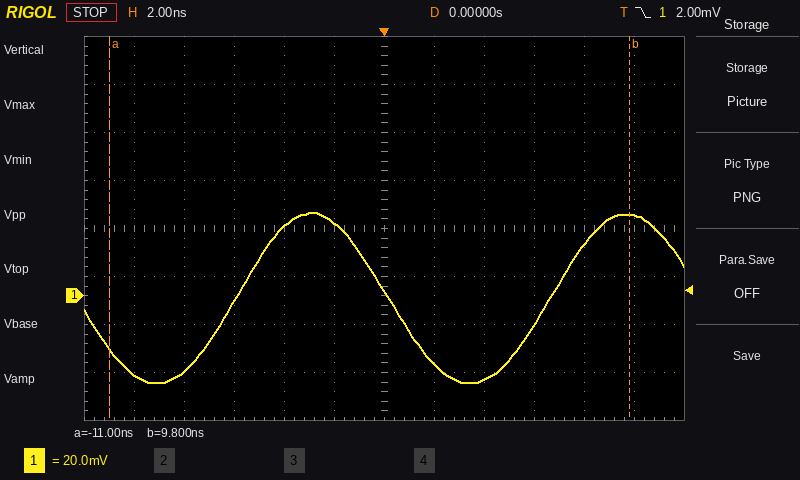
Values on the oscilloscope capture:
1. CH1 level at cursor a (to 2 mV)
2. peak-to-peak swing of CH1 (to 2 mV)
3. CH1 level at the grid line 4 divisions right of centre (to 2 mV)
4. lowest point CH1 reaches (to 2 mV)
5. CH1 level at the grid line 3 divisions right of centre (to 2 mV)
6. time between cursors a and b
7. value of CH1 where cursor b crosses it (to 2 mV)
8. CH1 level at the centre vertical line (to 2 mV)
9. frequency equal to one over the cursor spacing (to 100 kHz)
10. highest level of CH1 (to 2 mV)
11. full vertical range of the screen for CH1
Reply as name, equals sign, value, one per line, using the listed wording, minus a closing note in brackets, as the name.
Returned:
CH1 level at cursor a = -22 mV
peak-to-peak swing of CH1 = 70 mV
CH1 level at the grid line 4 divisions right of centre = 22 mV
lowest point CH1 reaches = -36 mV
CH1 level at the grid line 3 divisions right of centre = -12 mV
time between cursors a and b = 20.8 ns
value of CH1 where cursor b crosses it = 34 mV
CH1 level at the centre vertical line = 2 mV
frequency equal to one over the cursor spacing = 48.1 MHz
highest level of CH1 = 34 mV
full vertical range of the screen for CH1 = 160 mV
